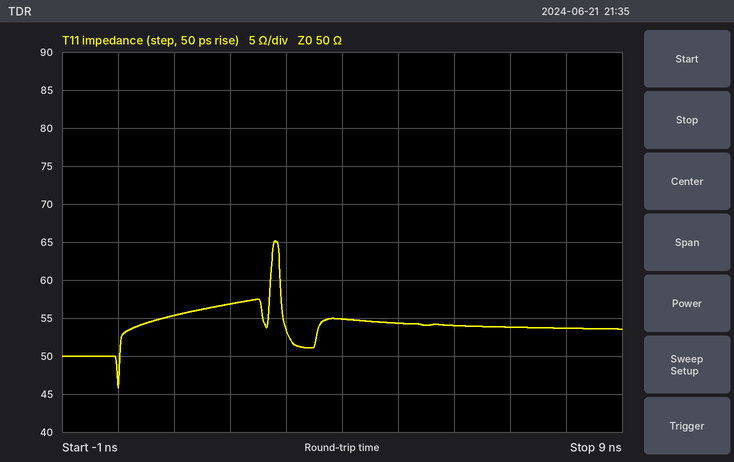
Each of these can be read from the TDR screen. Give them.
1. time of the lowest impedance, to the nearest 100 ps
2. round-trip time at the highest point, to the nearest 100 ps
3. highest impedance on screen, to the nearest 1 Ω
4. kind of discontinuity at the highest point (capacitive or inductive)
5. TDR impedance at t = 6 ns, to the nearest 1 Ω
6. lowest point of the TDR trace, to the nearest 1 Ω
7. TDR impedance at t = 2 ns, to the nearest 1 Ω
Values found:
0.0 ns
2.8 ns
65 Ω
inductive
54 Ω
46 Ω
57 Ω
